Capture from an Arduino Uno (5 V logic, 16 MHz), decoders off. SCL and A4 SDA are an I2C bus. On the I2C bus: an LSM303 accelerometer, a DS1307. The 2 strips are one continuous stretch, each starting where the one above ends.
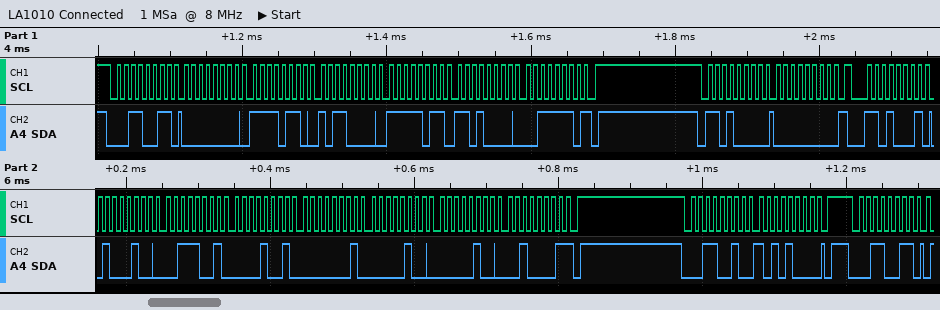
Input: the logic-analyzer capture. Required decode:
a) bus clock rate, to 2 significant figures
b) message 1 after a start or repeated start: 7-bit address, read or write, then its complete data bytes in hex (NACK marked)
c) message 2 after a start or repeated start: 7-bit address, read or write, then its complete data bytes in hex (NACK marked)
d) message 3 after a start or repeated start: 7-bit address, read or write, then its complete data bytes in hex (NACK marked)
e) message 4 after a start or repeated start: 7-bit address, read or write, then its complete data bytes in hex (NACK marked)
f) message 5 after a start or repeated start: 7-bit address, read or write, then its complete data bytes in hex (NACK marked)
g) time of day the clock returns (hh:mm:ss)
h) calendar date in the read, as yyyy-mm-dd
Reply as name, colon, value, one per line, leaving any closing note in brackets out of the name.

bus clock rate, to 2 significant figures: 100 kHz
message 1 after a start or repeated start: 7-bit address, read or write, then its complete data bytes in hex: 0x19 read: 00 F6 B0 FB D0 3E NACK
message 2 after a start or repeated start: 7-bit address, read or write, then its complete data bytes in hex: 0x68 write: 00
message 3 after a start or repeated start: 7-bit address, read or write, then its complete data bytes in hex: 0x68 read: 44 39 09 01 04 04 21 NACK
message 4 after a start or repeated start: 7-bit address, read or write, then its complete data bytes in hex: 0x19 write: A8
message 5 after a start or repeated start: 7-bit address, read or write, then its complete data bytes in hex: 0x19 read
time of day the clock returns: 09:39:44
calendar date in the read, as yyyy-mm-dd: 2021-04-04
